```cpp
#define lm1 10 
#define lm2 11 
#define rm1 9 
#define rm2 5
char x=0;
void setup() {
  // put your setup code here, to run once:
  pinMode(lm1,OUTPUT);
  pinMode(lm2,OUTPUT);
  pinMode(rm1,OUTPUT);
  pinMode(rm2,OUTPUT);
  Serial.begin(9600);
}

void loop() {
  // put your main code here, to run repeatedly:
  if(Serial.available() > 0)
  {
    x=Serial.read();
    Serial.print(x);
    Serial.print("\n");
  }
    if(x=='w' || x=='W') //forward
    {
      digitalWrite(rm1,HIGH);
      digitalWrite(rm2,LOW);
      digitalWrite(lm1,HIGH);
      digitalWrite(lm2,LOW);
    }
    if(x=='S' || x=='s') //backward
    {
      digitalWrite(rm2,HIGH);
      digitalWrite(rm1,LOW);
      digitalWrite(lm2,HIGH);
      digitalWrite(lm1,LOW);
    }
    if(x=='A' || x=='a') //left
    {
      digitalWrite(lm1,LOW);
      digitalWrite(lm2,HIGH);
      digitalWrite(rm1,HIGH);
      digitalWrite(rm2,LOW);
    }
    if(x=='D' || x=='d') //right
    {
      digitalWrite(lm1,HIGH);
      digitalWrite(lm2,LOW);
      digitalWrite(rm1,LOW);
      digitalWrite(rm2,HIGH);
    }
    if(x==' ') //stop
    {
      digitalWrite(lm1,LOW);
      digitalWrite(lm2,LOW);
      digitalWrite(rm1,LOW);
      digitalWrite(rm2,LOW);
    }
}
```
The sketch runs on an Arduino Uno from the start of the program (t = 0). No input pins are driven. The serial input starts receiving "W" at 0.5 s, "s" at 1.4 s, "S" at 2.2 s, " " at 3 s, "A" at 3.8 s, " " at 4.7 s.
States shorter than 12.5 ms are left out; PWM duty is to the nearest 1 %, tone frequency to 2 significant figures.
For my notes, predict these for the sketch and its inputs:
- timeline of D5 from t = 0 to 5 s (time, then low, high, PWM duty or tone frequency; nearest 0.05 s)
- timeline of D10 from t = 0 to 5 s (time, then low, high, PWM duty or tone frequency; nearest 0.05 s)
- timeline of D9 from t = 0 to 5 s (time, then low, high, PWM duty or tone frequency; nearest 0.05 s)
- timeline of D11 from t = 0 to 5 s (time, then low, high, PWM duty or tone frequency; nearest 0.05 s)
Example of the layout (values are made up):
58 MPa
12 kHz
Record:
0 s low; 1.4 s high; 3 s low
0 s low; 0.5 s high; 1.4 s low
0 s low; 0.5 s high; 1.4 s low; 3.8 s high; 4.7 s low
0 s low; 1.4 s high; 3 s low; 3.8 s high; 4.7 s low
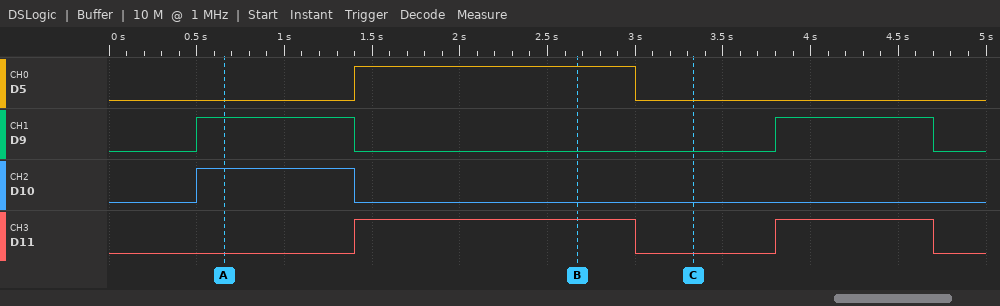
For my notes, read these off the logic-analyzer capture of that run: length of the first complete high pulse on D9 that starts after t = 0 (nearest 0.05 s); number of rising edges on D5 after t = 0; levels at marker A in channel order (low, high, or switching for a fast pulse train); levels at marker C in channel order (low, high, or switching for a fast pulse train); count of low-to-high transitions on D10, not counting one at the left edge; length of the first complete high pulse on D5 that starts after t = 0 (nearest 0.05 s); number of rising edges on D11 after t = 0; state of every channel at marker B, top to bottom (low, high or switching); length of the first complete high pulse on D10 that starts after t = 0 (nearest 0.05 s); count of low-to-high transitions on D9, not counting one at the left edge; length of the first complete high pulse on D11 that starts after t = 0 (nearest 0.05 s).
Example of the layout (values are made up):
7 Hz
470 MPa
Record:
0.90 s
1
D5 low, D9 high, D10 high, D11 low
D5 low, D9 low, D10 low, D11 low
1
1.60 s
2
D5 high, D9 low, D10 low, D11 high
0.90 s
2
1.60 s
